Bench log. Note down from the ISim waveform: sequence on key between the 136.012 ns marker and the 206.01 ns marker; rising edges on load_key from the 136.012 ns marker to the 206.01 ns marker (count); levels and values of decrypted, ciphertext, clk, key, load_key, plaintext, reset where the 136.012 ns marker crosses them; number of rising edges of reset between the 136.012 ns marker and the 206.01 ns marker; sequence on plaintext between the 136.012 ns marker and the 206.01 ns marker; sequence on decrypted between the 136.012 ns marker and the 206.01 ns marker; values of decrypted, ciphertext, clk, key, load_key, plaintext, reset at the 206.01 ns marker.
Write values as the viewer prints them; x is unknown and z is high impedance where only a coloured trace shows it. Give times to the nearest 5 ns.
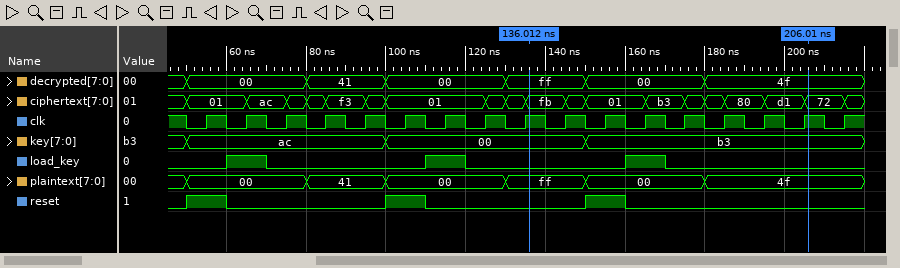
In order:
00, b3
1
decrypted=ff, ciphertext=fb, clk=1, key=00, load_key=0, plaintext=ff, reset=0
1
ff, 00, 4f
ff, 00, 4f
decrypted=4f, ciphertext=72, clk=1, key=b3, load_key=0, plaintext=4f, reset=0
